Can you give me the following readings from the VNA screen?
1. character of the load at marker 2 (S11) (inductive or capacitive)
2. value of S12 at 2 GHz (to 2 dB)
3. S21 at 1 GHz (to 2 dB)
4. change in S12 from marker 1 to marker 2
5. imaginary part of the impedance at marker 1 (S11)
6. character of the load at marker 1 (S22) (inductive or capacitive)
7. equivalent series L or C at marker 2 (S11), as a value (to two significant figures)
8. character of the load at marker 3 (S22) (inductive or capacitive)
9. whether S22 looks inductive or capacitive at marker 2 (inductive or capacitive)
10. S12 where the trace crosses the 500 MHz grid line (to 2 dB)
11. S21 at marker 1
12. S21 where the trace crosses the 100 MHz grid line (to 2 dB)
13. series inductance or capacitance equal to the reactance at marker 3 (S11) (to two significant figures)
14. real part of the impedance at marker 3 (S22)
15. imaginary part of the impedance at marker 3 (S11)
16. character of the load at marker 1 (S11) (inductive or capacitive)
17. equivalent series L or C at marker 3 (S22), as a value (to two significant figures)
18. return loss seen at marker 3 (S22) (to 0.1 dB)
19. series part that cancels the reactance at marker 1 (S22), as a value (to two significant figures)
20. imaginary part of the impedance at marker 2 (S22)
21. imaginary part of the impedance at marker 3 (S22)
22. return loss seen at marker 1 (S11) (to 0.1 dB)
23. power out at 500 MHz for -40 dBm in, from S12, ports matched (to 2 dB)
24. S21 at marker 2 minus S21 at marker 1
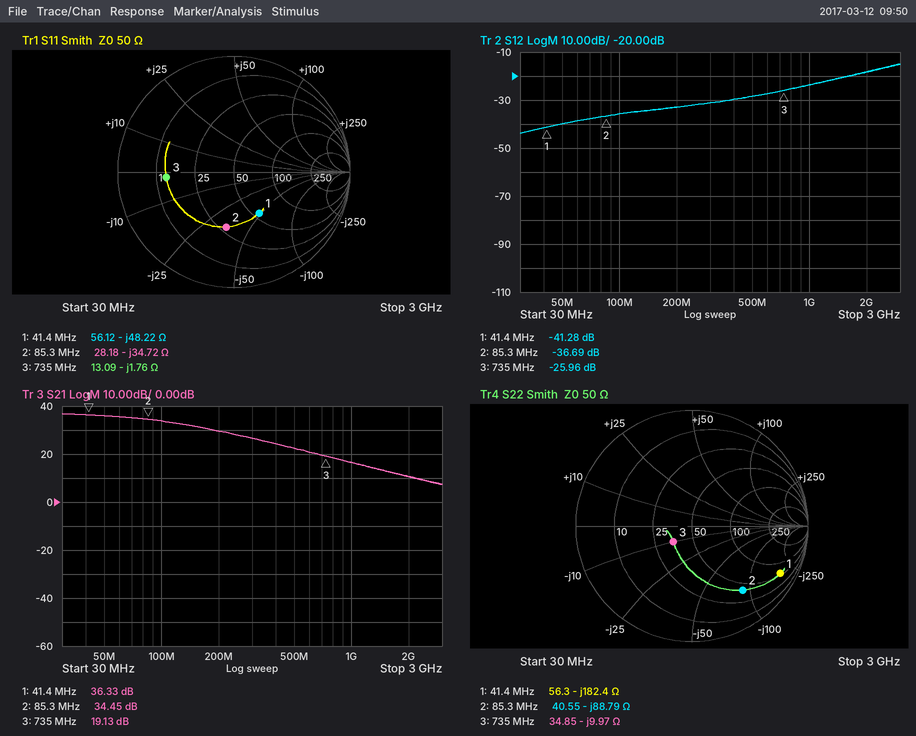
capacitive
-18 dB
16 dB
4.59 dB
-48.22 Ω
capacitive
54 pF
capacitive
capacitive
-28 dB
36.33 dB
34 dB
120 pF
34.85 Ω
-1.76 Ω
capacitive
22 pF
13.5 dB
700 nH
-88.79 Ω
-9.97 Ω
7.6 dB
-68 dBm
-1.88 dB
